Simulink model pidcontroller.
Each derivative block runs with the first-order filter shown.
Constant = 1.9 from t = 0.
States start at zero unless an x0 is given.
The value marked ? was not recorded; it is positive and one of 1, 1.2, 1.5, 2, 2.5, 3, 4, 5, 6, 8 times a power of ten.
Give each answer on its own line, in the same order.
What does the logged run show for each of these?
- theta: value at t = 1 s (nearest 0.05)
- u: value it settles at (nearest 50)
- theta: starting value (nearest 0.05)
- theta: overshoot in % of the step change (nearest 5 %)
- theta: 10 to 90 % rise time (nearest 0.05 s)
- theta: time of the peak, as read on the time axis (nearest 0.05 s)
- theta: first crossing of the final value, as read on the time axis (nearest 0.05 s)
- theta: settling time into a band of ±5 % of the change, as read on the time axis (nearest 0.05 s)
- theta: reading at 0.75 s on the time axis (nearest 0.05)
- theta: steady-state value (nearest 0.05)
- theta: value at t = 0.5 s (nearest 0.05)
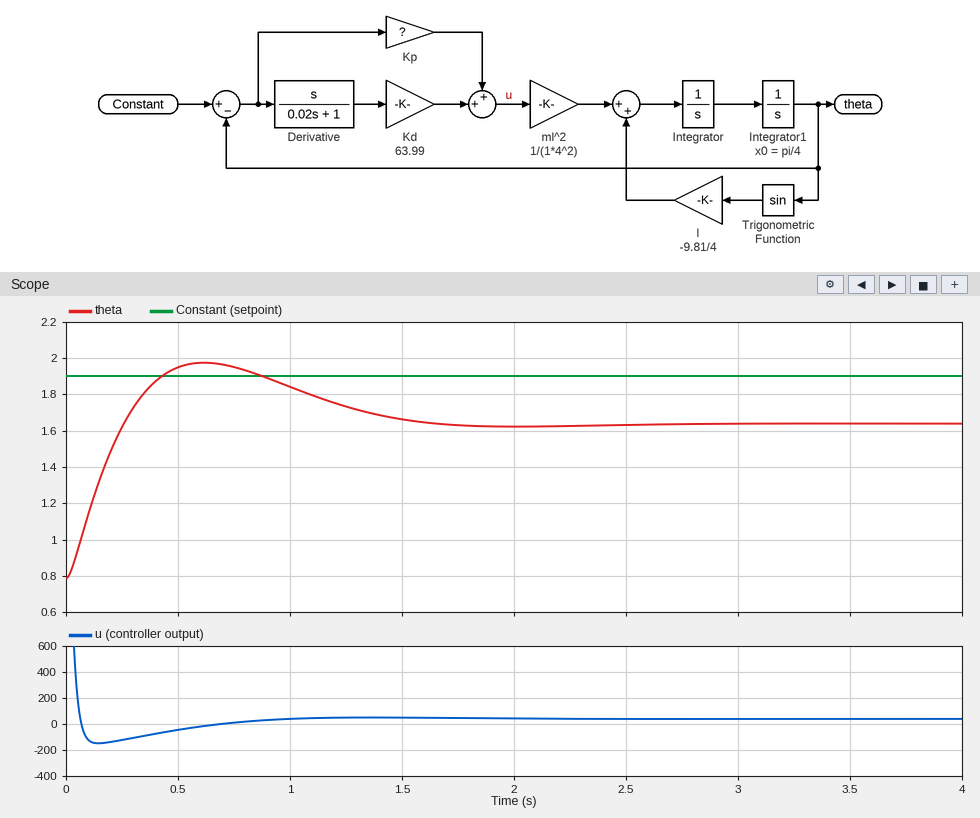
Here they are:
1.85
50
0.80
40 %
0.20 s
0.60 s
0.25 s
1.40 s
1.95
1.65
1.95
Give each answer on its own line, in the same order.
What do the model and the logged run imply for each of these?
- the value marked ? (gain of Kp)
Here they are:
150
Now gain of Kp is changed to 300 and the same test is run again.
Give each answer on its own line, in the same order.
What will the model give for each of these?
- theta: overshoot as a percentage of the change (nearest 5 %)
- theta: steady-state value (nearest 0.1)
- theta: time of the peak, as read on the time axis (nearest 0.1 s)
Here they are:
40 %
1.8
0.5 s
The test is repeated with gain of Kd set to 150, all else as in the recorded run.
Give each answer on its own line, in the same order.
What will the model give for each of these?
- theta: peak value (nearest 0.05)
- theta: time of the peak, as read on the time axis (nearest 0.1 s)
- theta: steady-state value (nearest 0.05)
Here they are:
1.90
0.4 s
1.65
